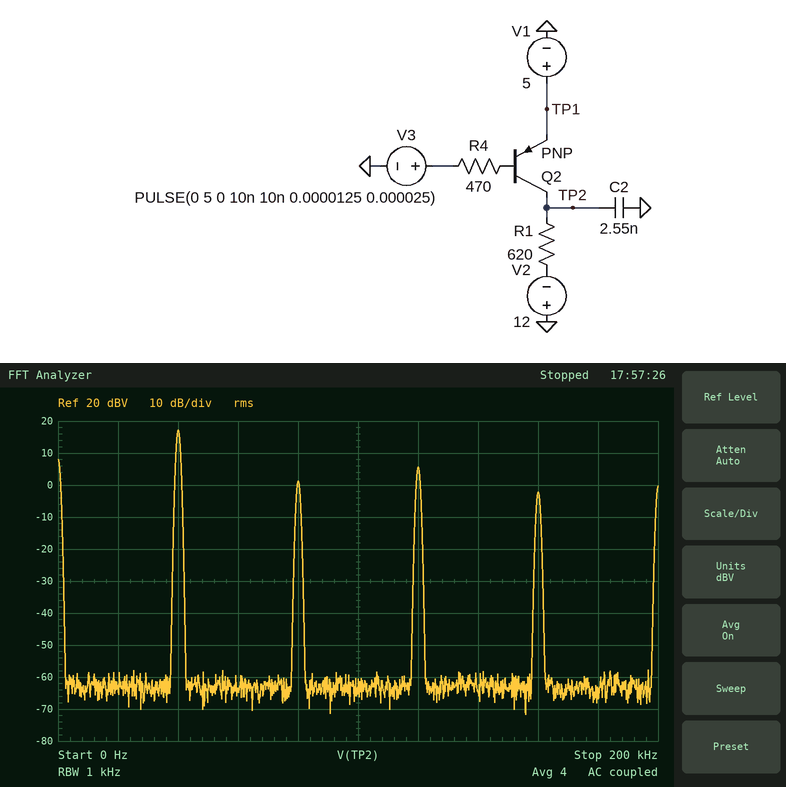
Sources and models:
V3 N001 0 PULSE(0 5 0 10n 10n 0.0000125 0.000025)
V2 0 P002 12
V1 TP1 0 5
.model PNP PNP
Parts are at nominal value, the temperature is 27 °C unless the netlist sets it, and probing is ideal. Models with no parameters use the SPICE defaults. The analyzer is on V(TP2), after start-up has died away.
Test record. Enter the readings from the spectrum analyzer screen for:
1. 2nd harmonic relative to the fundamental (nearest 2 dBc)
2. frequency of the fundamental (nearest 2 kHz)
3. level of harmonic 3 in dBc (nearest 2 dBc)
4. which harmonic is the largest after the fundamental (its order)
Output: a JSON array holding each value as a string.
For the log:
["-16 dBc", "40 kHz", "-12 dBc", "3"]
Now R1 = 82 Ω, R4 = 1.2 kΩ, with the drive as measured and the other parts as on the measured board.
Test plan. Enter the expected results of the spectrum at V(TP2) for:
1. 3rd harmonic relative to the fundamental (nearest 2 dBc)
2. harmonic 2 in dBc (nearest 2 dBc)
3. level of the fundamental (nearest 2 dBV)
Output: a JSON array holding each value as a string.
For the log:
["-10 dBc", "-36 dBc", "18 dBV"]
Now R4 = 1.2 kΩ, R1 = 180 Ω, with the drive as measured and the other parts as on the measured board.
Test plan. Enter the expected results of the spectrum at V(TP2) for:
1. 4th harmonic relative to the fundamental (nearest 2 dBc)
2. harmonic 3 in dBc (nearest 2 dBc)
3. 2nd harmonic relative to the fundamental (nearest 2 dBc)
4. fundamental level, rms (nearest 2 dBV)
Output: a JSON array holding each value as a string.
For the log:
["-28 dBc", "-10 dBc", "-26 dBc", "18 dBV"]
